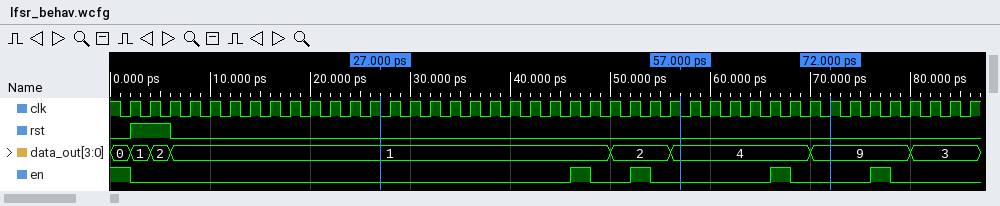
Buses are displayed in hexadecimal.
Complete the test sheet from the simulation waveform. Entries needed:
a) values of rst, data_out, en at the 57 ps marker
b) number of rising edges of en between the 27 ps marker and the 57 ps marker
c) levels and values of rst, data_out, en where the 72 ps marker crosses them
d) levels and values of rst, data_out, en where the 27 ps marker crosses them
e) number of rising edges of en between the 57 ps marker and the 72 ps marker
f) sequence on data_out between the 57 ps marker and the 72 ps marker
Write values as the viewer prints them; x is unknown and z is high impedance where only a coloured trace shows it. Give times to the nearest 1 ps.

rst=0, data_out=4, en=0
2
rst=0, data_out=9, en=0
rst=0, data_out=1, en=0
1
4, 9
